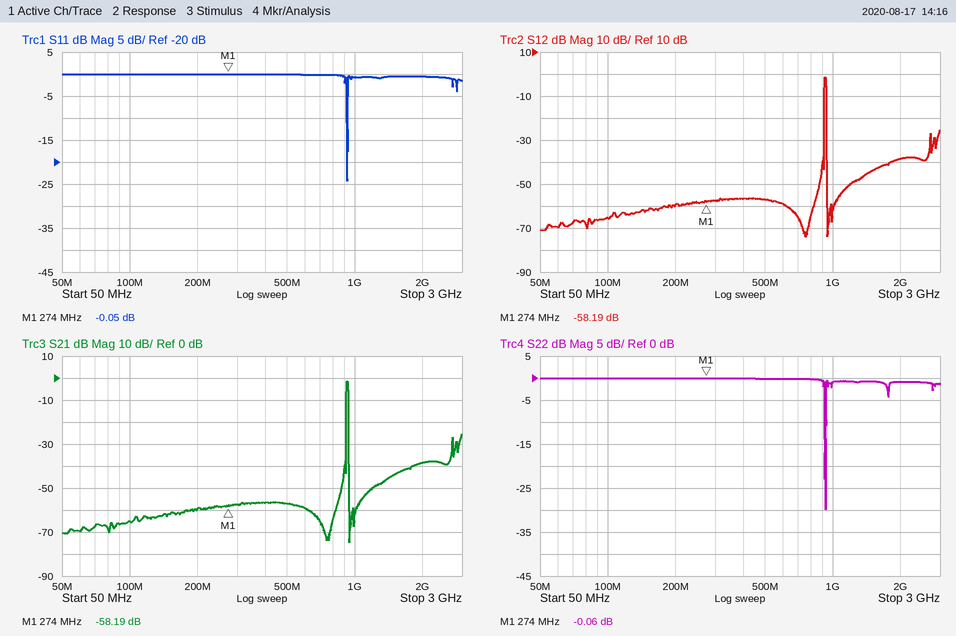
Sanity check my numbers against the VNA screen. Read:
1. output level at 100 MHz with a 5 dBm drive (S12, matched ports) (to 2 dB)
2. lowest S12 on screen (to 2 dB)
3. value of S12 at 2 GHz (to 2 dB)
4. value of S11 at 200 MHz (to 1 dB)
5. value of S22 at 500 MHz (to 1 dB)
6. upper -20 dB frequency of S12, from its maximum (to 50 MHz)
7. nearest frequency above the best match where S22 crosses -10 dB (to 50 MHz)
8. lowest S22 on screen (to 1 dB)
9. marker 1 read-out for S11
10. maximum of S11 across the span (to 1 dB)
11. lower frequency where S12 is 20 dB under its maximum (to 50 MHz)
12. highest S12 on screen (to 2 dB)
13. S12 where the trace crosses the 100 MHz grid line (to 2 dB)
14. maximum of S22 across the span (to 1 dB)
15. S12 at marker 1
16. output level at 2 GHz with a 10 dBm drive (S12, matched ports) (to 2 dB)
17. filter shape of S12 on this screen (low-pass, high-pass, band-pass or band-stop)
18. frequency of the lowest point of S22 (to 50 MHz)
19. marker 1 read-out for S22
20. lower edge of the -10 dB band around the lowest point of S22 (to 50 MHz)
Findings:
-60 dBm
-74 dB
-38 dB
0 dB
0 dB
950 MHz
950 MHz
-30 dB
-0.05 dB
0 dB
900 MHz
-2 dB
-66 dB
0 dB
-58.19 dB
-28 dBm
band-pass
950 MHz
-0.06 dB
900 MHz
